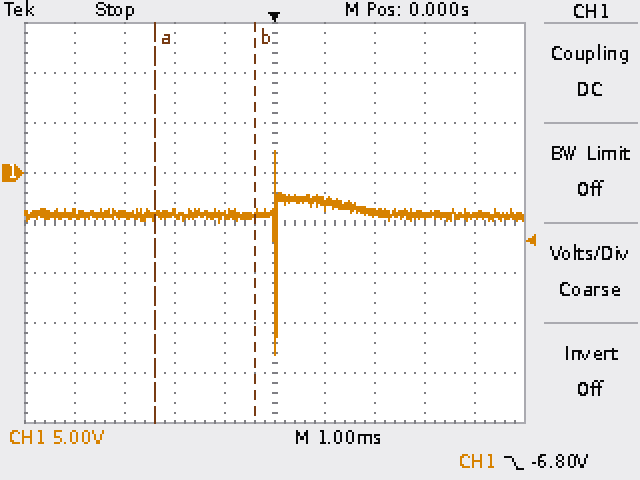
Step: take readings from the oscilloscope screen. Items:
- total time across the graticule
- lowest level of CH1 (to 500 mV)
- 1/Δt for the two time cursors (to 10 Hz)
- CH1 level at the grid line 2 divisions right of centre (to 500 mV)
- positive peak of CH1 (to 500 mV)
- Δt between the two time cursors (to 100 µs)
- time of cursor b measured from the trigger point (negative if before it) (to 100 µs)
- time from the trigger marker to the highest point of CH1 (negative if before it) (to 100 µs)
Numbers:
10 ms
-18.0 V
500 Hz
-4.0 V
2.0 V
2.0 ms
-400 µs
0.0 ms
